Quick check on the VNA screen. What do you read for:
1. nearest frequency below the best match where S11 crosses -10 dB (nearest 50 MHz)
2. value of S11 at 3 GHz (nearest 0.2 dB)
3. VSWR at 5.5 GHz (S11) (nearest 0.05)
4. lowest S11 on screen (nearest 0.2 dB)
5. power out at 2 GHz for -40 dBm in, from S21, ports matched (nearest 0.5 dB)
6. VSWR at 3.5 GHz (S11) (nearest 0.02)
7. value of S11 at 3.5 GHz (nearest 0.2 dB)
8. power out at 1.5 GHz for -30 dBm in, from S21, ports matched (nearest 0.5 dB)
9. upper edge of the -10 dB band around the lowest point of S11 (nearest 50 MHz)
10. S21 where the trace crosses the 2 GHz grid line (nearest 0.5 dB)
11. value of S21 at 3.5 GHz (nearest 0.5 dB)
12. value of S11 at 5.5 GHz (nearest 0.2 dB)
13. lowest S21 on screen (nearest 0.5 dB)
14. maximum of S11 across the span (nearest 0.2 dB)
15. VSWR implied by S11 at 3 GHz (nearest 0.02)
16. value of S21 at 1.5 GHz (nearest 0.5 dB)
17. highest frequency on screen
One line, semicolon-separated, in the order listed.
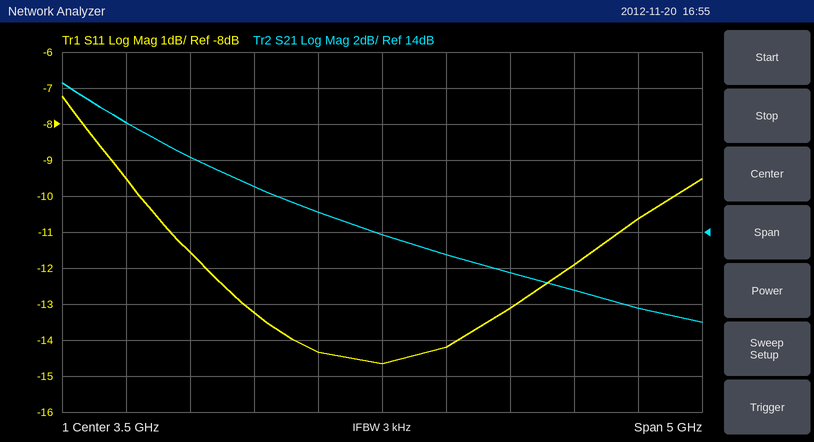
1.60 GHz; -14.4 dB; 1.85; -14.6 dB; -22.0 dBm; 1.46; -14.6 dB; -10.0 dBm; 5.80 GHz; 18.0 dB; 14.0 dB; -10.6 dB; 9.0 dB; -7.2 dB; 1.48; 20.0 dB; 6 GHz
